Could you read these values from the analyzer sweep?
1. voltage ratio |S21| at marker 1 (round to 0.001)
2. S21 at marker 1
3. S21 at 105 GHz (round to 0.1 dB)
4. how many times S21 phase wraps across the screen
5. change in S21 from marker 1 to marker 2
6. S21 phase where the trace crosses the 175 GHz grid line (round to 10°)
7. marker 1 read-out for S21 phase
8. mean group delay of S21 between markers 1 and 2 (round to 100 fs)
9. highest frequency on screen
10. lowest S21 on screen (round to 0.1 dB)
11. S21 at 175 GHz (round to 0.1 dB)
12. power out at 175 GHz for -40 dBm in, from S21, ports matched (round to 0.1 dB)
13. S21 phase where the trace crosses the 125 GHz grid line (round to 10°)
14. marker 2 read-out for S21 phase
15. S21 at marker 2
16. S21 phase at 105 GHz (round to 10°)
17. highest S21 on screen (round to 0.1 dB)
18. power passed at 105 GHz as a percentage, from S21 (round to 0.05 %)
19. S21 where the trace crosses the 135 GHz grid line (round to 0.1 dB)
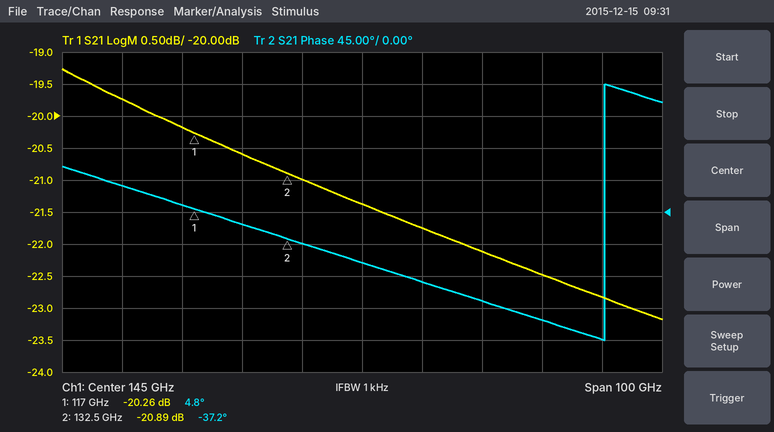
0.097
-20.26 dB
-19.7 dB
1
-0.63 dB
-150°
4.8°
7.5 ps
195 GHz
-23.2 dB
-22.5 dB
-62.5 dBm
-20°
-37.2°
-20.89 dB
40°
-19.3 dB
1.05 %
-21.0 dB
